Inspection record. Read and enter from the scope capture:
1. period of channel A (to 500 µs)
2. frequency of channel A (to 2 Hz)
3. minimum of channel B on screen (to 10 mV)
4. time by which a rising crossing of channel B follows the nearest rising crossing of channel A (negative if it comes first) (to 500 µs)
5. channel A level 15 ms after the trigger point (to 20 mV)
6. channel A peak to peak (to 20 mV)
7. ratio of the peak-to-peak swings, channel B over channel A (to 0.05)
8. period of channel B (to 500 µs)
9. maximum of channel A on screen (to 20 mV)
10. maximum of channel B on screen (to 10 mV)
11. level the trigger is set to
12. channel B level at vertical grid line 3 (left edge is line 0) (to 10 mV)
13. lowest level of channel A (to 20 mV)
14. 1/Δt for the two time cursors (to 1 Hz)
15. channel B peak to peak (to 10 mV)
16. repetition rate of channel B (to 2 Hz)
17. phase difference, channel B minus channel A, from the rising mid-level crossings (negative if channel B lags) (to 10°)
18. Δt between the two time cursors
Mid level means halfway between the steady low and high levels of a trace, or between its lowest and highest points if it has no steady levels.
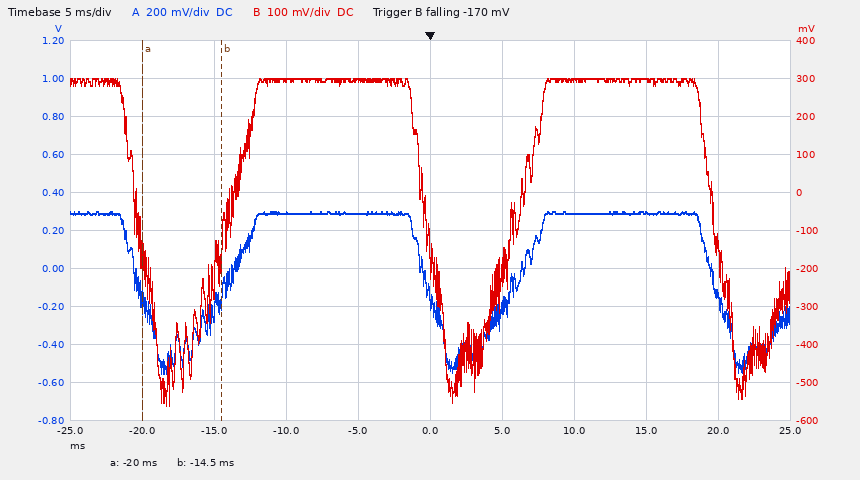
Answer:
20.0 ms
50 Hz
-560 mV
0.0 ms
300 mV
860 mV
1.00
20.0 ms
300 mV
300 mV
-170 mV
300 mV
-560 mV
182 Hz
860 mV
50 Hz
0°
5.5 ms
